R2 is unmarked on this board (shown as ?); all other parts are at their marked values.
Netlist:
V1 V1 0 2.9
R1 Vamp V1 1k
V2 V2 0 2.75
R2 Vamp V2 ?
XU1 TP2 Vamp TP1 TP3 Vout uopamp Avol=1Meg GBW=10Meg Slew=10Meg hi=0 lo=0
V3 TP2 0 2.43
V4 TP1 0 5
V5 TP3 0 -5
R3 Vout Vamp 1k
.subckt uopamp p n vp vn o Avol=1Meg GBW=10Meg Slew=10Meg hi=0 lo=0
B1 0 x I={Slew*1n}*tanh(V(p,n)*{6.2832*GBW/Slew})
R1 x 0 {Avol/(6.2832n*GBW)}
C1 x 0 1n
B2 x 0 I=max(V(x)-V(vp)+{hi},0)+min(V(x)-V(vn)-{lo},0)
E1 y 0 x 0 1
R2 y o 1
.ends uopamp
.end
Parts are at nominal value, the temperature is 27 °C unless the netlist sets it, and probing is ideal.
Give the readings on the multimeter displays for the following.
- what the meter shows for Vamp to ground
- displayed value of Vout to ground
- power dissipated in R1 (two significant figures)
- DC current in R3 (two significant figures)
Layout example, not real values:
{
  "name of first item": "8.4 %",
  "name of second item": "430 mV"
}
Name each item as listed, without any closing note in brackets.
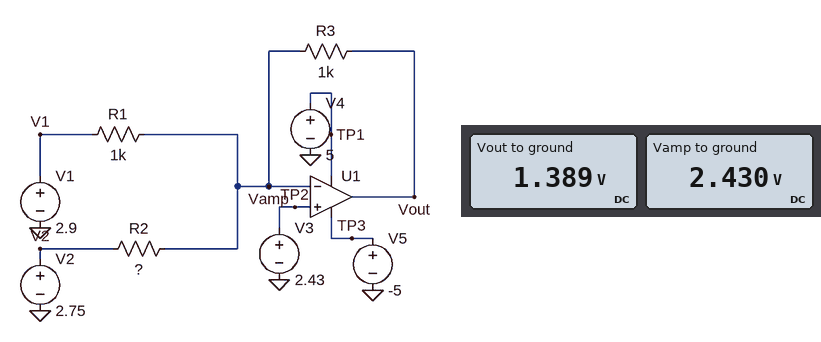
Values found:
{
  "what the meter shows for Vamp to ground": "2.430 V",
  "displayed value of Vout to ground": "1.389 V",
  "power dissipated in R1": "220 µW",
  "DC current in R3": "1.0 mA"
}
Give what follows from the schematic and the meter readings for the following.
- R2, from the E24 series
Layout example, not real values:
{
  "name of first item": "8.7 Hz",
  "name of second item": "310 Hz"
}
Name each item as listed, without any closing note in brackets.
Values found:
{
  "R2, from the E24 series": "560 Ω"
}
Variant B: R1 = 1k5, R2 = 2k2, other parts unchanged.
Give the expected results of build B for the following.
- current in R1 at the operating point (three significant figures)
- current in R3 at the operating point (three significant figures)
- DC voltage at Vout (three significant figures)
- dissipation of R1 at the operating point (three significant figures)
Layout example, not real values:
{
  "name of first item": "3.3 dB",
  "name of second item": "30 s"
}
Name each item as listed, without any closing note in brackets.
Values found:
{
  "current in R1 at the operating point": "313 µA",
  "current in R3 at the operating point": "459 µA",
  "DC voltage at Vout": "1.97 V",
  "dissipation of R1 at the operating point": "147 µW"
}
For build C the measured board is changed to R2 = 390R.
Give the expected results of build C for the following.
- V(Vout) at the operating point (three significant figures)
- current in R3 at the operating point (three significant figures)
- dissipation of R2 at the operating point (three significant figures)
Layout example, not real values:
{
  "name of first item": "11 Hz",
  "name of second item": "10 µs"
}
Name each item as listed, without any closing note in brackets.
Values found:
{
  "V(Vout) at the operating point": "1.14 V",
  "current in R3 at the operating point": "1.29 mA",
  "dissipation of R2 at the operating point": "263 µW"
}
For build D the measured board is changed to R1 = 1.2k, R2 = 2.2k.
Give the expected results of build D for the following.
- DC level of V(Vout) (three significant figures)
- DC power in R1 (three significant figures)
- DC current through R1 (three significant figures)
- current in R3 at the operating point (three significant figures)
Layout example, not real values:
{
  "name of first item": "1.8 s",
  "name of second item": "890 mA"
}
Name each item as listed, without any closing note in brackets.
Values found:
{
  "DC level of V(Vout)": "1.89 V",
  "DC power in R1": "184 µW",
  "DC current through R1": "392 µA",
  "current in R3 at the operating point": "537 µA"
}
